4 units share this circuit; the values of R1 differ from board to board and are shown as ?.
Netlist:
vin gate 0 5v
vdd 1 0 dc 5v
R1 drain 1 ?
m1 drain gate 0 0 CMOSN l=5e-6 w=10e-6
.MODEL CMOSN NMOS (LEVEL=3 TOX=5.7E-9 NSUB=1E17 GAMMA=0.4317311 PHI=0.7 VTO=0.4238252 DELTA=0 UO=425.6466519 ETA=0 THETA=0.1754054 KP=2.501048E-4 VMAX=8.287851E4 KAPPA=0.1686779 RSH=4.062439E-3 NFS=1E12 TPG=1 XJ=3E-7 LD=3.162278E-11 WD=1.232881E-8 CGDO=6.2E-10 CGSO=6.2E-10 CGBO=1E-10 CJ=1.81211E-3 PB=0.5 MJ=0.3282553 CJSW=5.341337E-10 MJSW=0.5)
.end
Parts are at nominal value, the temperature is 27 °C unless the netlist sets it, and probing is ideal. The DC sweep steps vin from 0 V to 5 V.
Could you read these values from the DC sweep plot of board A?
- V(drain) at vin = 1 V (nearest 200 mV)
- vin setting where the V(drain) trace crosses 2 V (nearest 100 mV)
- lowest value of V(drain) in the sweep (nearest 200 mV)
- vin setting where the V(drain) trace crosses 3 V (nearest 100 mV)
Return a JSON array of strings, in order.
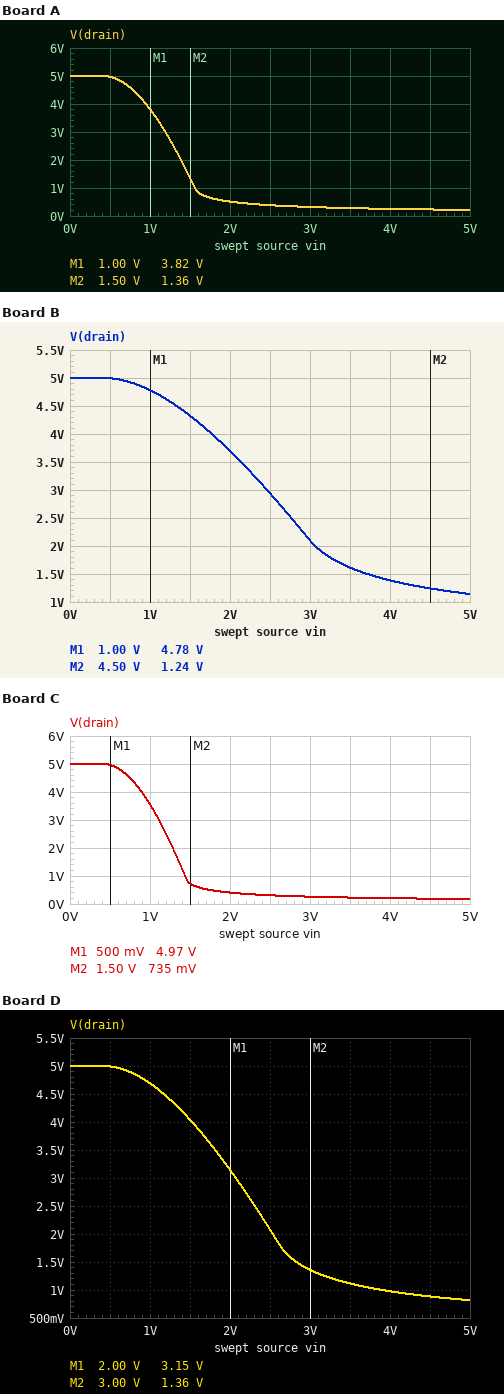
["3.8 V", "1.4 V", "200 mV", "1.2 V"]
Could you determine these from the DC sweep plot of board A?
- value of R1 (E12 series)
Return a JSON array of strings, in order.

["18 kΩ"]
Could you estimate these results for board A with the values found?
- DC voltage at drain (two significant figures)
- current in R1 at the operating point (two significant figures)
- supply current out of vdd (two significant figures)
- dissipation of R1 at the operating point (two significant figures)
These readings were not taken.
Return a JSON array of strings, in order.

["220 mV", "270 µA", "270 µA", "1.3 mW"]
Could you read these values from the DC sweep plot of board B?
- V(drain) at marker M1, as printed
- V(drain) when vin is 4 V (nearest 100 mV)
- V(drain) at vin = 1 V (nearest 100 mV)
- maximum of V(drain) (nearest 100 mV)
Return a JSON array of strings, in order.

["4.78 V", "1.4 V", "4.8 V", "5.0 V"]
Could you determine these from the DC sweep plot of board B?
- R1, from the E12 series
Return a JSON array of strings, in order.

["3.3 kΩ"]
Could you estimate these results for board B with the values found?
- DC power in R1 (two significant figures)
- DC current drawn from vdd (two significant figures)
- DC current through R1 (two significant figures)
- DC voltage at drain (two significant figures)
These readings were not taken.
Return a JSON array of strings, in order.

["4.5 mW", "1.2 mA", "1.2 mA", "1.1 V"]
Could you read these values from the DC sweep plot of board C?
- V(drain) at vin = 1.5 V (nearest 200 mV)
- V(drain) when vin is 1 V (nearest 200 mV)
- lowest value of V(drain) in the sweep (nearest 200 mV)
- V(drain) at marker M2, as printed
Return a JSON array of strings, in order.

["800 mV", "3.6 V", "200 mV", "735 mV"]
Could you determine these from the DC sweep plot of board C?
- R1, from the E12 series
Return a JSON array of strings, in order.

["22 kΩ"]
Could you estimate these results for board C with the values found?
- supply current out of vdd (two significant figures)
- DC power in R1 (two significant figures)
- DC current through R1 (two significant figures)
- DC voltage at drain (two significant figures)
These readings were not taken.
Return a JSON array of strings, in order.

["220 µA", "1.1 mW", "220 µA", "180 mV"]
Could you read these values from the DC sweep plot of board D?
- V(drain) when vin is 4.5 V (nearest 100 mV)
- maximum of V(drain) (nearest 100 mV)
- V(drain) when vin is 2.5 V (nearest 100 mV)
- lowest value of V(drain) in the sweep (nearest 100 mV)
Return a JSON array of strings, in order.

["900 mV", "5.0 V", "2.1 V", "800 mV"]
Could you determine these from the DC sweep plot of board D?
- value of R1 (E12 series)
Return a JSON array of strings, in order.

["4.7 kΩ"]
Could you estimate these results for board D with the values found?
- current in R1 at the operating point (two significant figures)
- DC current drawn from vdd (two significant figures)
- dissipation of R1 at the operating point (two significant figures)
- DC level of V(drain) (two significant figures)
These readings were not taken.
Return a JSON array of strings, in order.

["890 µA", "890 µA", "3.7 mW", "820 mV"]
